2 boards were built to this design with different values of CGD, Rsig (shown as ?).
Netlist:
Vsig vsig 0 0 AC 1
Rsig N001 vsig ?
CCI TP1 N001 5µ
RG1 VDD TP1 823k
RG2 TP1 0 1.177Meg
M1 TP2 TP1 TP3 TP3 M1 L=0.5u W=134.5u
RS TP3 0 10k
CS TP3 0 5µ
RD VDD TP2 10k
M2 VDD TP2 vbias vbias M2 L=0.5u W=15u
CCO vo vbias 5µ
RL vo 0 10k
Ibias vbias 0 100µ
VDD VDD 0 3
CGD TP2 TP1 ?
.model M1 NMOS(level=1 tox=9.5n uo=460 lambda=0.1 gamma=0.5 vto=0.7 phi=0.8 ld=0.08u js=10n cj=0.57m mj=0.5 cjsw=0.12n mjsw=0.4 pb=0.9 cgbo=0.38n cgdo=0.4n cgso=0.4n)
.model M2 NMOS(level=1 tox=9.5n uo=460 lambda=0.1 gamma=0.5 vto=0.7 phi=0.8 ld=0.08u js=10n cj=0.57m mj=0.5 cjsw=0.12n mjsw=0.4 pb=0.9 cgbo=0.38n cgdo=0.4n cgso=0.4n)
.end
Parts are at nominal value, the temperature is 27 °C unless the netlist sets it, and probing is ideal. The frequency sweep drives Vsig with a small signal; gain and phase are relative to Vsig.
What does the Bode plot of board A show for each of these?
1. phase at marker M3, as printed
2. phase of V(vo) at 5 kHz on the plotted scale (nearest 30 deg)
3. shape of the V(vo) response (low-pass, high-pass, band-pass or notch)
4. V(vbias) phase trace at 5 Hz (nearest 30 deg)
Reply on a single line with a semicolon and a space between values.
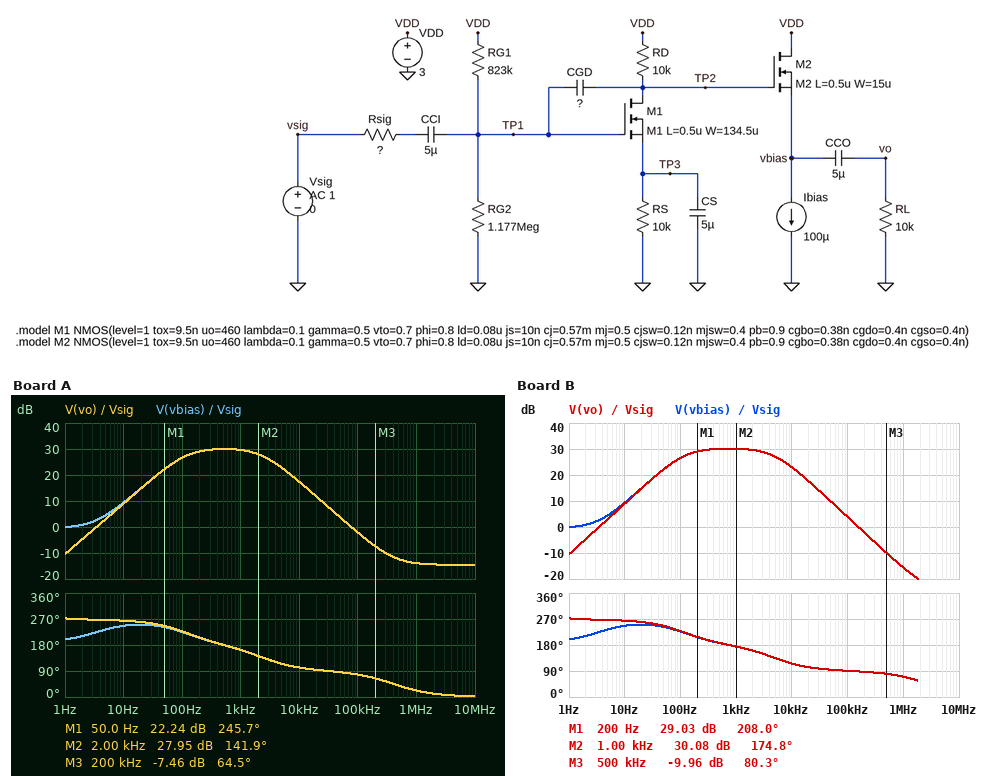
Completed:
64.5 deg; 120 deg; band-pass; 240 deg
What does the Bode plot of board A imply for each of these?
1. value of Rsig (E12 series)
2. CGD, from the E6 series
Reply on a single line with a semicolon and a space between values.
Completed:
1 kΩ; 1.5 nF
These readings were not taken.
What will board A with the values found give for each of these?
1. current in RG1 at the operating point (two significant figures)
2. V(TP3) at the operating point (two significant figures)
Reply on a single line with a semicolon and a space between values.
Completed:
1.5 µA; 1.0 V
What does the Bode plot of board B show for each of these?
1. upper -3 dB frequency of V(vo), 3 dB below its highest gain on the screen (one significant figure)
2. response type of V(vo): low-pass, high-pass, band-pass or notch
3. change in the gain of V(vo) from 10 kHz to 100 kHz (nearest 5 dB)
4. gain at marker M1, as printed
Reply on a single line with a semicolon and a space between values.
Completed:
5 kHz; band-pass; -20 dB; 29.03 dB
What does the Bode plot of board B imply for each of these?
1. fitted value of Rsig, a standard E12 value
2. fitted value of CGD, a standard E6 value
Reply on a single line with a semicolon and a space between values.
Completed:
3.9 kΩ; 220 pF
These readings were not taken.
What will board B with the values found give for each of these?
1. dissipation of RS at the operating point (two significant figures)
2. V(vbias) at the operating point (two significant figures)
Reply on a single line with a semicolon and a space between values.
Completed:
100 µW; 1.1 V
